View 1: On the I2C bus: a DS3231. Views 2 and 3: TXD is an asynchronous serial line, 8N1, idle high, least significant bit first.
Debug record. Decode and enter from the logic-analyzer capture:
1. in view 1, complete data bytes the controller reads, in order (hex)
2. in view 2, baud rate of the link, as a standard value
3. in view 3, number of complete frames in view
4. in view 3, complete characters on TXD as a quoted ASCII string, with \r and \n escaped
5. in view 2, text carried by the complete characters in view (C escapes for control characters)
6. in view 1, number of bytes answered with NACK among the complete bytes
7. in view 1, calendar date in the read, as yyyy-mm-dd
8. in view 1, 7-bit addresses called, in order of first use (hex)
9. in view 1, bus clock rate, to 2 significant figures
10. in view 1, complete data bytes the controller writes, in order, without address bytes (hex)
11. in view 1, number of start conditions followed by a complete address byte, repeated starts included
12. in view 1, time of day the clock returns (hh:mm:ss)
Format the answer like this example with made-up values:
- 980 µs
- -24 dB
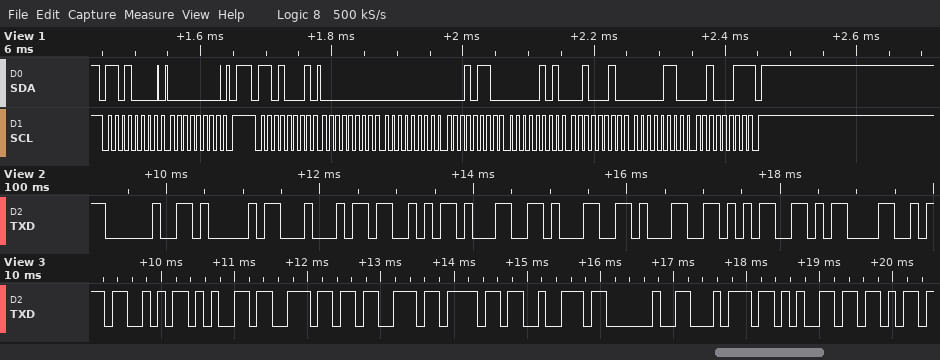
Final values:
- 00 00 16 05 22 06 23
- 9600 baud
- 10
- "Sensor tek"
- " ADS1115\r"
- 1
- 2023-06-22
- 0x68
- 100 kHz
- 00
- 2
- 16:00:00
